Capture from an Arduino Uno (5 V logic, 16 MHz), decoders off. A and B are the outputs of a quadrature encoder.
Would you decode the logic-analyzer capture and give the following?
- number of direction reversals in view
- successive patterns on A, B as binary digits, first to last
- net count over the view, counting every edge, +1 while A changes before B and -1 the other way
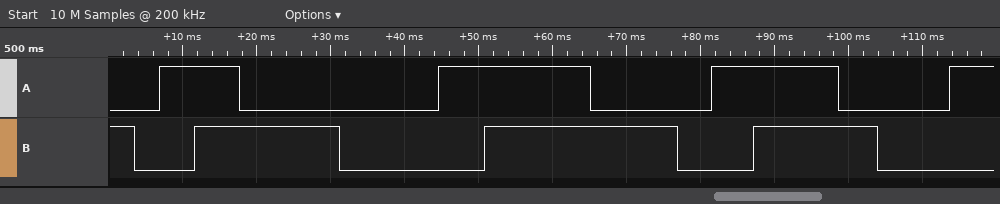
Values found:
0
01 00 10 11 01 00 10 11 01 00 10 11 01 00 10
+14
